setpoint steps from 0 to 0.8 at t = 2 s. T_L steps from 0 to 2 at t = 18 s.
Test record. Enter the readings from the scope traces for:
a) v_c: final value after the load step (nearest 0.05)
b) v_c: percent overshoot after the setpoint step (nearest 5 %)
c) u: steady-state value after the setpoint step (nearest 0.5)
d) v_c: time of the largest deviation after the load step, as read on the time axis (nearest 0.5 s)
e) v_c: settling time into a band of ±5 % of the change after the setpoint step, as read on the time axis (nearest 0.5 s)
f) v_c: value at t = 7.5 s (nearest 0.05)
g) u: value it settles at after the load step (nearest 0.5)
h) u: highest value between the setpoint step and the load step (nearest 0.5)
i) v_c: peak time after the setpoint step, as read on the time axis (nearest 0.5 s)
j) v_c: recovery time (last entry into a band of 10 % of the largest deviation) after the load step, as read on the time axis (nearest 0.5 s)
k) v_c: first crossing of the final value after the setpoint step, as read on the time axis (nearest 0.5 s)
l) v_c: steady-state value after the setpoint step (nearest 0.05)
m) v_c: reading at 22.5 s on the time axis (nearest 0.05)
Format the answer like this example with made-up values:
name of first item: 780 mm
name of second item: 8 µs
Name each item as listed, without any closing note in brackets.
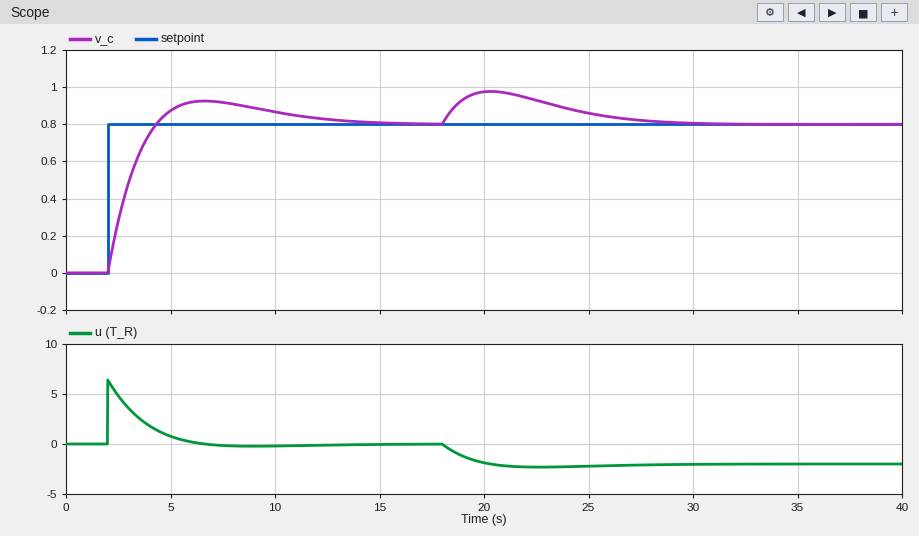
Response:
v_c: final value after the load step: 0.80
v_c: percent overshoot after the setpoint step: 15 %
u: steady-state value after the setpoint step: 0.0
v_c: time of the largest deviation after the load step, as read on the time axis: 20.5 s
v_c: settling time into a band of ±5 % of the change after the setpoint step, as read on the time axis: 11.5 s
v_c: value at t = 7.5 s: 0.90
u: value it settles at after the load step: -2.0
u: highest value between the setpoint step and the load step: 6.5
v_c: peak time after the setpoint step, as read on the time axis: 6.5 s
v_c: recovery time (last entry into a band of 10 % of the largest deviation) after the load step, as read on the time axis: 28.0 s
v_c: first crossing of the final value after the setpoint step, as read on the time axis: 4.5 s
v_c: steady-state value after the setpoint step: 0.80
v_c: reading at 22.5 s on the time axis: 0.95
